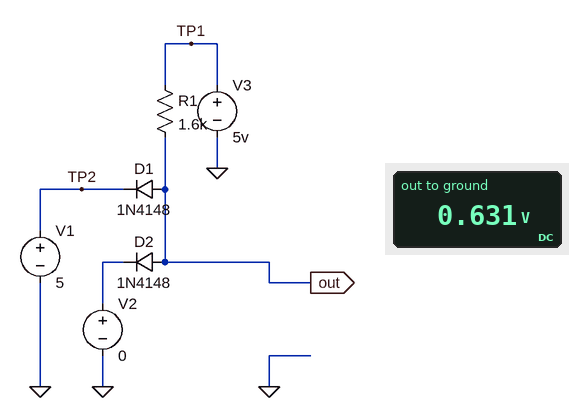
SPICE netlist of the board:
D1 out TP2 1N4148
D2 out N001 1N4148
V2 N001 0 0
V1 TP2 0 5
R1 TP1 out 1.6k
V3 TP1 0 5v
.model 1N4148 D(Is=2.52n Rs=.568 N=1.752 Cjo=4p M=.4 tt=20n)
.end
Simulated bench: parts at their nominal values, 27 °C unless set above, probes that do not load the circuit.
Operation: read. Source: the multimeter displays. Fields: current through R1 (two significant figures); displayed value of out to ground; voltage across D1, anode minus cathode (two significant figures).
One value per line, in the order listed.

2.7 mA
0.631 V
-4.4 V
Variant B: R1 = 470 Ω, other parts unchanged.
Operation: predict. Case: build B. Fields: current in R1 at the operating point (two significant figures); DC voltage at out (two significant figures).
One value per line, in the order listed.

9.2 mA
690 mV
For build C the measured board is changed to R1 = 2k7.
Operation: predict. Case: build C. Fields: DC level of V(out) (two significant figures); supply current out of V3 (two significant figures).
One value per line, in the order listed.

610 mV
1.6 mA
